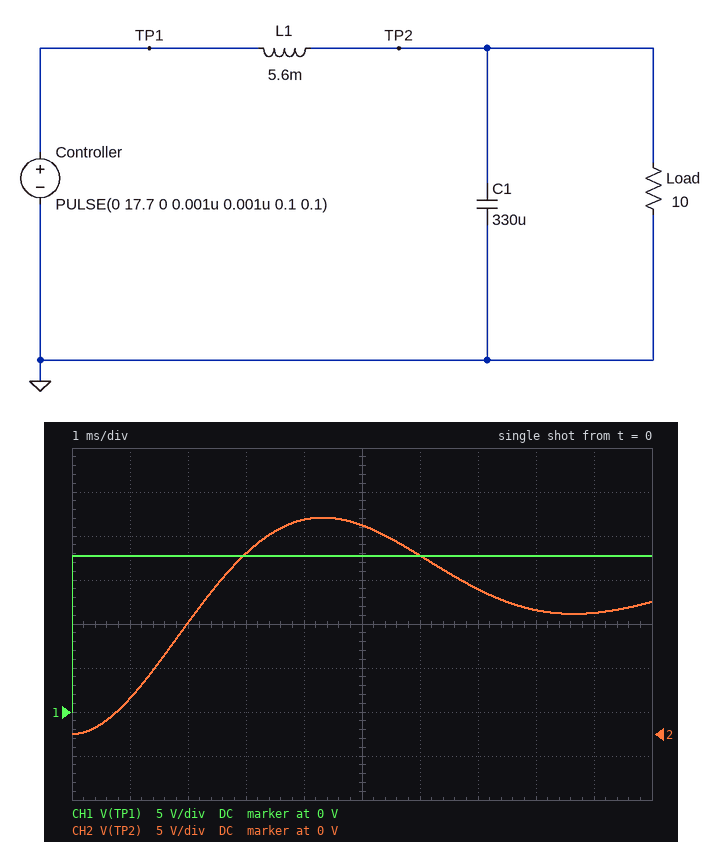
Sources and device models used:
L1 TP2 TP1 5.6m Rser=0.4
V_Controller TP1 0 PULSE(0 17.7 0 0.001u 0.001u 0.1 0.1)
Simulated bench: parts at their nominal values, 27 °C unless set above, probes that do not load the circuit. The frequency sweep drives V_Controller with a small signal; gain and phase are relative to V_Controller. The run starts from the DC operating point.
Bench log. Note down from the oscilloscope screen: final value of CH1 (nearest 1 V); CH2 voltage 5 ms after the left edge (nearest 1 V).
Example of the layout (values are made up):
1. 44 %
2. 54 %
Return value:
1. 18 V
2. 24 V
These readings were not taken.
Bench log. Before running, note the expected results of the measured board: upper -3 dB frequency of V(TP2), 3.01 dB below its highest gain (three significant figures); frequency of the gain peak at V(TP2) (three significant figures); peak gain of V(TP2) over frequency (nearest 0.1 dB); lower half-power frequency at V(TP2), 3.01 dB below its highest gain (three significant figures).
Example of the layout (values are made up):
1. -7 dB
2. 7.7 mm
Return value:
1. 139 Hz
2. 112 Hz
3. 6.0 dB
4. 74.8 Hz
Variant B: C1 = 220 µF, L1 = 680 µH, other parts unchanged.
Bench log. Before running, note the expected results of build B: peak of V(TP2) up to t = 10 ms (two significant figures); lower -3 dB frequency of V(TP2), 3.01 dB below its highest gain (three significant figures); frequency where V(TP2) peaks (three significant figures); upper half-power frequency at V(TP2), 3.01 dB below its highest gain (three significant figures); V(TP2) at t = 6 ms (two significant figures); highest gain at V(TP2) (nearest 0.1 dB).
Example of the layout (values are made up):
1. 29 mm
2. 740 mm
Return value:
1. 26 V
2. 307 Hz
3. 403 Hz
4. 480 Hz
5. 18 V
6. 7.9 dB
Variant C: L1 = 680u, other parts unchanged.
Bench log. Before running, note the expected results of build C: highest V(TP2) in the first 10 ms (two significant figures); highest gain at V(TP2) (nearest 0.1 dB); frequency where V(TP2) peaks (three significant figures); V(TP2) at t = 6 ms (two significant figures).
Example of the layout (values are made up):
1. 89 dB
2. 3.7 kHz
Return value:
1. 26 V
2. 7.5 dB
3. 328 Hz
4. 16 V
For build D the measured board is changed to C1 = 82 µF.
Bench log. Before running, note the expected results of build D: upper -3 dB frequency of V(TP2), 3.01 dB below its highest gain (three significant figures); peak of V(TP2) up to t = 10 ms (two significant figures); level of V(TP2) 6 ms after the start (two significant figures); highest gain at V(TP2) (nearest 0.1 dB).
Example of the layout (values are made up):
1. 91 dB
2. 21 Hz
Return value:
1. 284 Hz
2. 21 V
3. 17 V
4. 1.9 dB
